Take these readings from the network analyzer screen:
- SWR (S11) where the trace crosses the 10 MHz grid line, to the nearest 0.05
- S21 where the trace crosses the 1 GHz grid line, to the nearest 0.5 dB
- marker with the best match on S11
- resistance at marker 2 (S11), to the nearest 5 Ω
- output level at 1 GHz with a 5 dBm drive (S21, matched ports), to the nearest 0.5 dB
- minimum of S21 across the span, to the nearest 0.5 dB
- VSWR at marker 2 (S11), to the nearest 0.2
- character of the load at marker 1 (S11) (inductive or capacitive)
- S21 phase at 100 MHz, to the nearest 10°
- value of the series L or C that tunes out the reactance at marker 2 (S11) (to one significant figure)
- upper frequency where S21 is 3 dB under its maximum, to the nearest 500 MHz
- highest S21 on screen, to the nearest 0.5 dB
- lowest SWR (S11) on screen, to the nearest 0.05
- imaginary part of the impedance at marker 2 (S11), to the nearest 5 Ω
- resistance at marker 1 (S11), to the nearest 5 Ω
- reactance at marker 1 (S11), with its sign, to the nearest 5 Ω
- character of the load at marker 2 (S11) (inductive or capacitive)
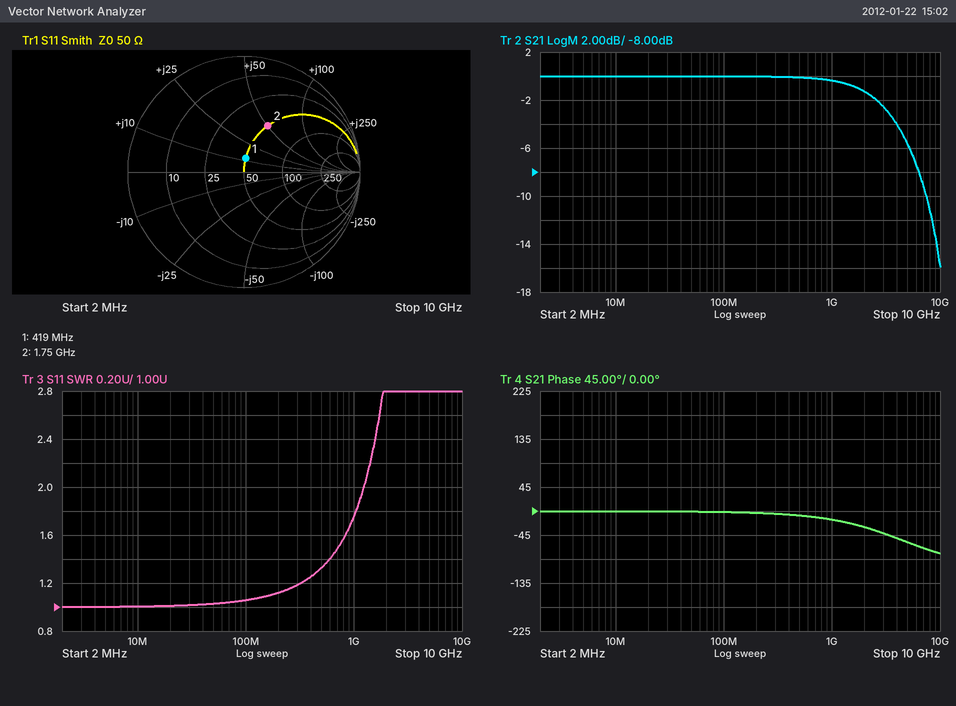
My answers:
1.00
-0.5 dB
marker 1
50 Ω
4.5 dBm
-16.0 dB
2.6
inductive
0°
2 pF
3.5 GHz
0.0 dB
1.00
+50 Ω
50 Ω
+10 Ω
inductive
